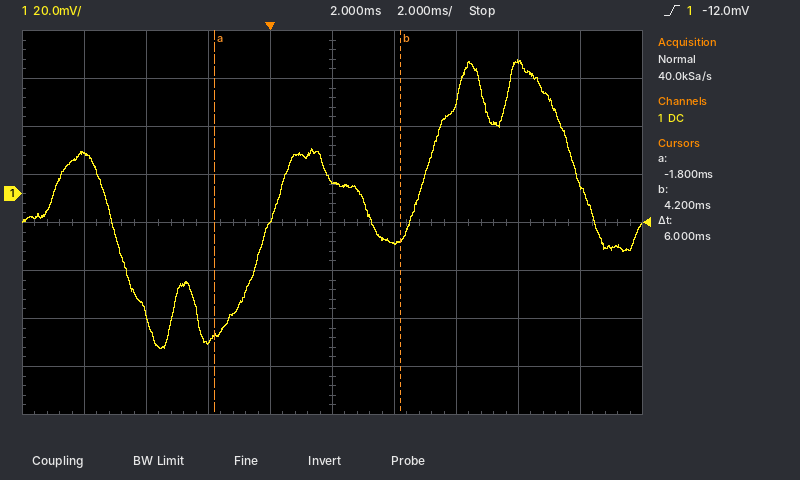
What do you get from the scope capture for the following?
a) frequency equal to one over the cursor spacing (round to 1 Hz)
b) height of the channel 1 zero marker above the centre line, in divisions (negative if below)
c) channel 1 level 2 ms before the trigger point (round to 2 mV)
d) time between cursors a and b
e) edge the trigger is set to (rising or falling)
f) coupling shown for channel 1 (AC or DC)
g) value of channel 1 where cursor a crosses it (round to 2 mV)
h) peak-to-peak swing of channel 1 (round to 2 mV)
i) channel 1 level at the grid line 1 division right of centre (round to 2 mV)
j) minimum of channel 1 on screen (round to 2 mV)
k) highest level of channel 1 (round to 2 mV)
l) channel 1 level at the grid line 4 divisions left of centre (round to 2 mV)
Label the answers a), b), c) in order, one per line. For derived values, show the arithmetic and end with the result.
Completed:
a) 1 / 6 ms ≈ 167 Hz
b) +0.6 div
c) -62 mV
d) 6 ms
e) rising
f) DC
g) -60 mV
h) 56 mV − (-64 mV) = 120 mV
i) -20 mV
j) -64 mV
k) 56 mV
l) 16 mV
